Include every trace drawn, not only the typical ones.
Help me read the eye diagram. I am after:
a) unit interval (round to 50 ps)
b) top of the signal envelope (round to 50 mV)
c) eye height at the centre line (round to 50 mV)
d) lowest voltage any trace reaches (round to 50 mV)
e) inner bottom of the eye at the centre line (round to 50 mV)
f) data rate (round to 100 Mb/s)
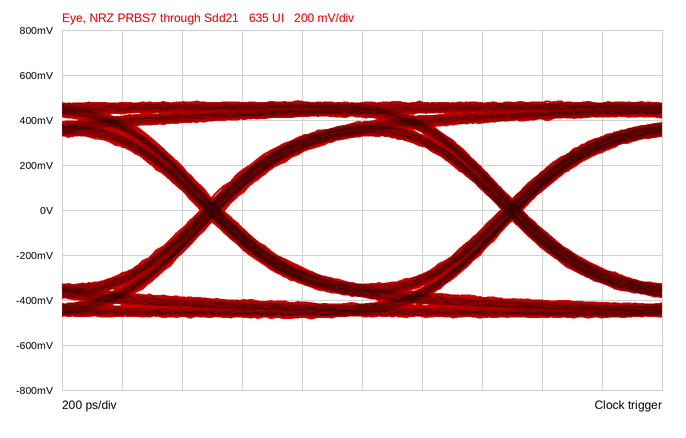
1.00 ns
500 mV
650 mV
-500 mV
-350 mV
1.0 Gb/s
